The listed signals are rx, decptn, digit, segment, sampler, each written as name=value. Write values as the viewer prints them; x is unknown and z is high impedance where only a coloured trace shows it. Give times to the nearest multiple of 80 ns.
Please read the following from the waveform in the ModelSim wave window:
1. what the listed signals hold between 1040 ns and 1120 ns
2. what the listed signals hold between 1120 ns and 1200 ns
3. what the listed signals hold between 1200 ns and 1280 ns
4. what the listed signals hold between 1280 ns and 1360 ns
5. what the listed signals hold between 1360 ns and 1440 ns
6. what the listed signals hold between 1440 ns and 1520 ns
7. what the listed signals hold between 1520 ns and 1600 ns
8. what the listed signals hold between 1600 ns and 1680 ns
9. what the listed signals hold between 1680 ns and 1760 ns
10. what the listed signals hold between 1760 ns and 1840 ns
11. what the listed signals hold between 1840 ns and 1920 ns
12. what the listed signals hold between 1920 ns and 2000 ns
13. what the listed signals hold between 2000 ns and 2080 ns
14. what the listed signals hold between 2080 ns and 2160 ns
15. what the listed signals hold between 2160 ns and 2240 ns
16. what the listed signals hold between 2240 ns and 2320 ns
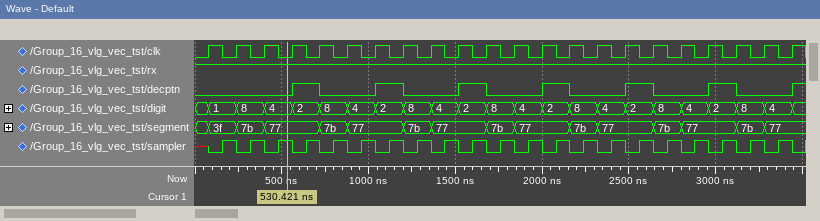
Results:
rx=1, decptn=1, digit=2, segment=77, sampler=0
rx=1, decptn=1, digit=2, segment=77, sampler=1
rx=1, decptn=0, digit=8, segment=7b, sampler=0
rx=1, decptn=0, digit=8, segment=7b, sampler=1
rx=1, decptn=0, digit=4, segment=77, sampler=0
rx=1, decptn=0, digit=4, segment=77, sampler=1
rx=1, decptn=1, digit=2, segment=77, sampler=0
rx=1, decptn=1, digit=2, segment=77, sampler=1
rx=1, decptn=0, digit=8, segment=7b, sampler=0
rx=1, decptn=0, digit=8, segment=7b, sampler=1
rx=1, decptn=0, digit=4, segment=77, sampler=0
rx=1, decptn=0, digit=4, segment=77, sampler=1
rx=1, decptn=1, digit=2, segment=77, sampler=0
rx=1, decptn=1, digit=2, segment=77, sampler=1
rx=1, decptn=0, digit=8, segment=7b, sampler=0
rx=1, decptn=0, digit=8, segment=7b, sampler=1
